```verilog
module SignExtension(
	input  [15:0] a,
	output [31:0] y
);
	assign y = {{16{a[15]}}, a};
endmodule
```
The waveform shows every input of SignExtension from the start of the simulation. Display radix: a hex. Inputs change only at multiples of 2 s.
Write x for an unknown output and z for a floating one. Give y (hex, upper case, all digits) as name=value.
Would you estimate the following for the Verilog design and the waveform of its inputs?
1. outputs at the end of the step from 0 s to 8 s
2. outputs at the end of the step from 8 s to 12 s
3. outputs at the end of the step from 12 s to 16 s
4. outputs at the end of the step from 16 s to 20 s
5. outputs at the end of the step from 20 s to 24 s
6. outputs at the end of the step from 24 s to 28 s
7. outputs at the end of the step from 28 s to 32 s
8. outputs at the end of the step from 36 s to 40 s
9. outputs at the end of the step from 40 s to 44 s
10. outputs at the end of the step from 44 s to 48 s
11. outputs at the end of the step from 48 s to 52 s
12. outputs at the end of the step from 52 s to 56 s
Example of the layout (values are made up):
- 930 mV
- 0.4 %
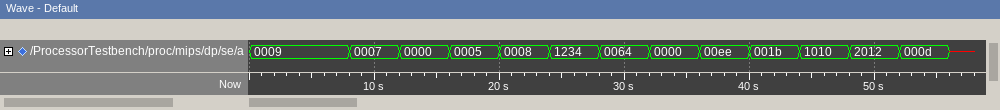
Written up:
- y=00000009
- y=00000007
- y=00000000
- y=00000005
- y=00000008
- y=00001234
- y=00000064
- y=000000EE
- y=0000001B
- y=00001010
- y=00002012
- y=0000000D
